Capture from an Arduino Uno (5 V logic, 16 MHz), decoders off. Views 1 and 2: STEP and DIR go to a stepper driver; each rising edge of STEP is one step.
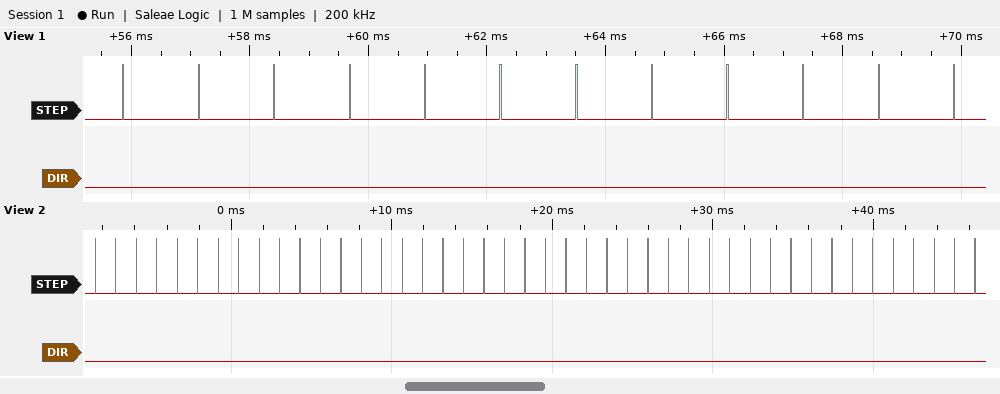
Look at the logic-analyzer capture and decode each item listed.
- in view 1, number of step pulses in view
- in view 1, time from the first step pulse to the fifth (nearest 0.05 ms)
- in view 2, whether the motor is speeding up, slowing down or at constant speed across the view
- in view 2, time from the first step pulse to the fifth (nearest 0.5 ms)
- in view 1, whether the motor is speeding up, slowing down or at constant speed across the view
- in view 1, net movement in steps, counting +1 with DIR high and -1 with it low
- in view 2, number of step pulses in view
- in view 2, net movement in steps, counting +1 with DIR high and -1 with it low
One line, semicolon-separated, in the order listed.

12; 5.10 ms; constant speed; 5.0 ms; constant speed; -12; 44; -44
